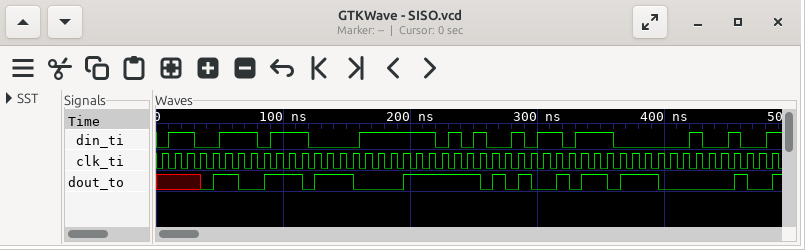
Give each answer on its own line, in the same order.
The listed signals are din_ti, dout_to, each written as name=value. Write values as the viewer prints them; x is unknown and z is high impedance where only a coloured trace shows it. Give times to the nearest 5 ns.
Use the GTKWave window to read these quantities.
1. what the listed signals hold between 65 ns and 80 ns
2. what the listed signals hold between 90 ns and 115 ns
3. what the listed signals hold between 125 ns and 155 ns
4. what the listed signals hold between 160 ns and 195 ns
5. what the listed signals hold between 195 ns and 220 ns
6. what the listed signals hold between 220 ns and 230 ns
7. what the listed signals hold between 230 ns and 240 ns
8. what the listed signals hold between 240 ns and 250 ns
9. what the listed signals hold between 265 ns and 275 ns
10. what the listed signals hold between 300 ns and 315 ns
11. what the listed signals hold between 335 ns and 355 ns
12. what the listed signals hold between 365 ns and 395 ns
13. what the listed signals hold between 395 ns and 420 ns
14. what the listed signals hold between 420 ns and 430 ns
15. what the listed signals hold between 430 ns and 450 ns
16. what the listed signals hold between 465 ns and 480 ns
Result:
din_ti=1, dout_to=0
din_ti=1, dout_to=1
din_ti=0, dout_to=1
din_ti=1, dout_to=0
din_ti=1, dout_to=1
din_ti=0, dout_to=1
din_ti=1, dout_to=1
din_ti=0, dout_to=1
din_ti=0, dout_to=1
din_ti=1, dout_to=0
din_ti=1, dout_to=1
din_ti=0, dout_to=1
din_ti=0, dout_to=0
din_ti=1, dout_to=0
din_ti=0, dout_to=0
din_ti=0, dout_to=0
